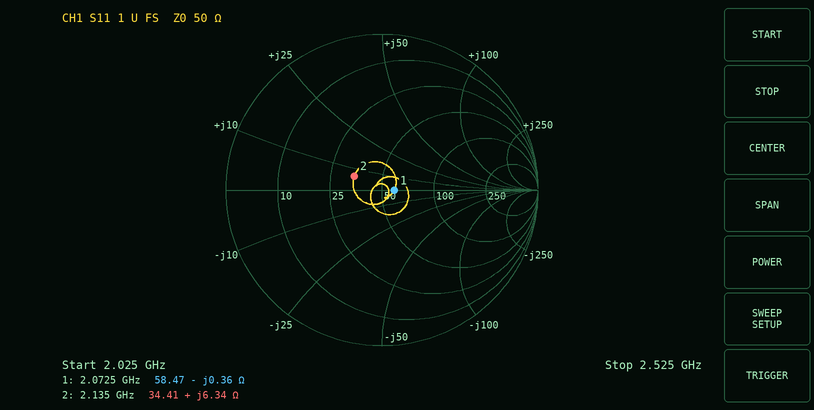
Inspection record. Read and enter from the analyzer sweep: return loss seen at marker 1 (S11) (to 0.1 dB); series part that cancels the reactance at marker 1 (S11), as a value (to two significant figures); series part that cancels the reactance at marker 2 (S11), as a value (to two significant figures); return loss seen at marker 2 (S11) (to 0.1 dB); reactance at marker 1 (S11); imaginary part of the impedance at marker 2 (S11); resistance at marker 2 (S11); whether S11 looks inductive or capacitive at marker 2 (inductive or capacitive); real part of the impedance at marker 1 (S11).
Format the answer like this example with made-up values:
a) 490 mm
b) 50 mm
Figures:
a) 22.1 dB
b) 28 pH
c) 12 pF
d) 14.0 dB
e) -0.36 Ω
f) +6.34 Ω
g) 34.41 Ω
h) inductive
i) 58.47 Ω
